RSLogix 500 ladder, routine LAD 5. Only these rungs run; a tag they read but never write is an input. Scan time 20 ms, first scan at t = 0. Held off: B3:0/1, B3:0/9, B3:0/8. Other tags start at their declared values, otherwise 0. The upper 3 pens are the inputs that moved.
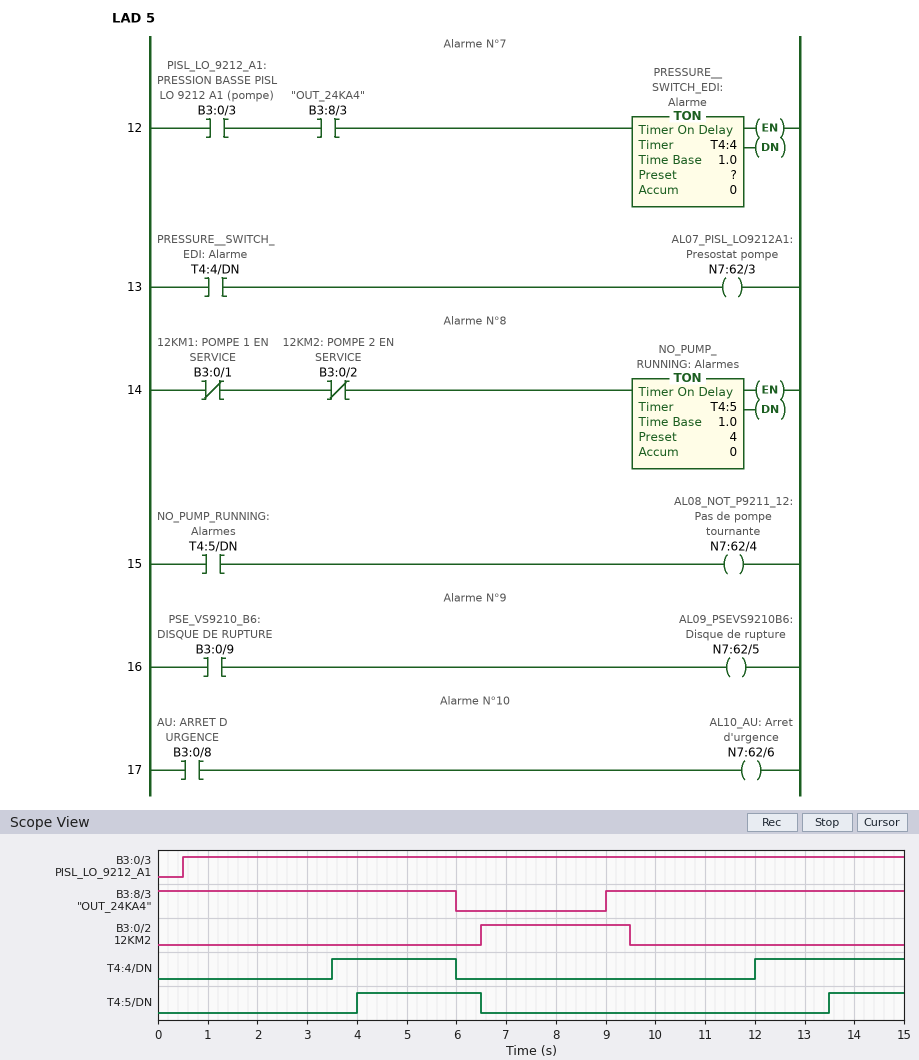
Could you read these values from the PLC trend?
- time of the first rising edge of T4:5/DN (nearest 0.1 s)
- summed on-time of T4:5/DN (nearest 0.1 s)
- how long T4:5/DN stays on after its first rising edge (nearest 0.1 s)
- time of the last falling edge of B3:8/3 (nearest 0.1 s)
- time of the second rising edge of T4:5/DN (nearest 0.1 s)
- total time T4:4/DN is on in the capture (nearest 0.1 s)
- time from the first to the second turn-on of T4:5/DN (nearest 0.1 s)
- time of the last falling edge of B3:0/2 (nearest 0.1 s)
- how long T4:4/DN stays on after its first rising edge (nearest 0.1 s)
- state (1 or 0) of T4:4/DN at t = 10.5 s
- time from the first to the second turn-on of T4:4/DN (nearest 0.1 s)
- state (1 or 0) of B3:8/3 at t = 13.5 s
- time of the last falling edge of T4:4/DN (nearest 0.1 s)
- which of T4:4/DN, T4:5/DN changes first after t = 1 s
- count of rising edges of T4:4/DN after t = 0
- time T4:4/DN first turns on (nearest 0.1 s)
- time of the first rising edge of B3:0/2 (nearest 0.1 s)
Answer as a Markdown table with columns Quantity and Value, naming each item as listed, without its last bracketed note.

| Quantity | Value |
|---|---|
| time of the first rising edge of T4:5/DN | 4.0 s |
| summed on-time of T4:5/DN | 4.0 s |
| how long T4:5/DN stays on after its first rising edge | 2.5 s |
| time of the last falling edge of B3:8/3 | 6.0 s |
| time of the second rising edge of T4:5/DN | 13.5 s |
| total time T4:4/DN is on in the capture | 5.5 s |
| time from the first to the second turn-on of T4:5/DN | 9.5 s |
| time of the last falling edge of B3:0/2 | 9.5 s |
| how long T4:4/DN stays on after its first rising edge | 2.5 s |
| state (1 or 0) of T4:4/DN at t = 10.5 s | 0 |
| time from the first to the second turn-on of T4:4/DN | 8.5 s |
| state (1 or 0) of B3:8/3 at t = 13.5 s | 1 |
| time of the last falling edge of T4:4/DN | 6.0 s |
| which of T4:4/DN, T4:5/DN changes first after t = 1 s | T4:4/DN |
| count of rising edges of T4:4/DN after t = 0 | 2 |
| time T4:4/DN first turns on | 3.5 s |
| time of the first rising edge of B3:0/2 | 6.5 s |
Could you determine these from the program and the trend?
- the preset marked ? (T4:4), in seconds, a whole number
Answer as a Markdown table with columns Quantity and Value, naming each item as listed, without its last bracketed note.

| Quantity | Value |
|---|---|
| the preset marked ? (T4:4), in seconds, a whole number | 3 s |
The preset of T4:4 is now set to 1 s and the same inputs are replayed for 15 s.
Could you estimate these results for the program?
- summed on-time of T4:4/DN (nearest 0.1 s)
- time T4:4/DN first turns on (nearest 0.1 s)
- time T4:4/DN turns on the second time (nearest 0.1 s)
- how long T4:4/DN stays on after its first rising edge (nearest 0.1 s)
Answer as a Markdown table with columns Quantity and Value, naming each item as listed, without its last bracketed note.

| Quantity | Value |
|---|---|
| summed on-time of T4:4/DN | 9.5 s |
| time T4:4/DN first turns on | 1.5 s |
| time T4:4/DN turns on the second time | 10.0 s |
| how long T4:4/DN stays on after its first rising edge | 4.5 s |
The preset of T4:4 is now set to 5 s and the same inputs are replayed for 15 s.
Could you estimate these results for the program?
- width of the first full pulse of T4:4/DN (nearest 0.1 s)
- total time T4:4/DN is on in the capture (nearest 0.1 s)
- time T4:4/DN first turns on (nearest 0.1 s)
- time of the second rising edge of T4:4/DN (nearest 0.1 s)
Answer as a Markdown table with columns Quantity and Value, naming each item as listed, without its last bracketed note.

| Quantity | Value |
|---|---|
| width of the first full pulse of T4:4/DN | 0.5 s |
| total time T4:4/DN is on in the capture | 1.5 s |
| time T4:4/DN first turns on | 5.5 s |
| time of the second rising edge of T4:4/DN | 14.0 s |
